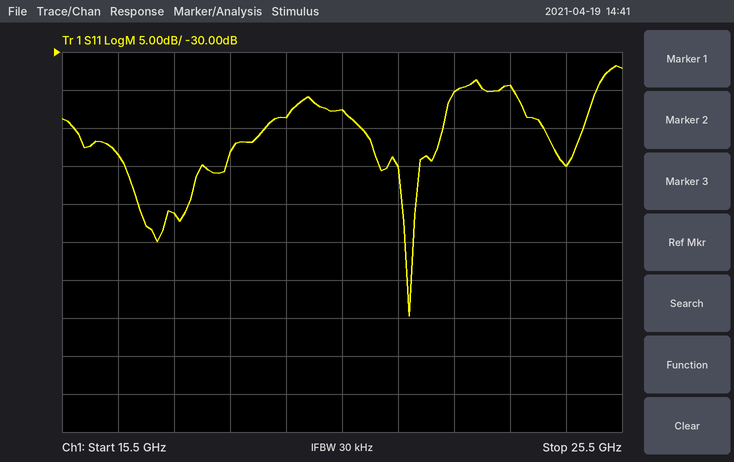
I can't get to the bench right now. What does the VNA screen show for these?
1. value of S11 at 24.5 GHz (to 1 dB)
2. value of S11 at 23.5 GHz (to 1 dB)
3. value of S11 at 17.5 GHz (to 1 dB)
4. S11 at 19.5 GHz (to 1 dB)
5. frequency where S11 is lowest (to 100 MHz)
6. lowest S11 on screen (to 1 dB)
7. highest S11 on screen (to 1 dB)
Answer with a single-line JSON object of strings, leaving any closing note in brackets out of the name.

{"value of S11 at 24.5 GHz": "-45 dB", "value of S11 at 23.5 GHz": "-34 dB", "value of S11 at 17.5 GHz": "-51 dB", "S11 at 19.5 GHz": "-39 dB", "frequency where S11 is lowest": "21.7 GHz", "lowest S11 on screen": "-65 dB", "highest S11 on screen": "-32 dB"}
